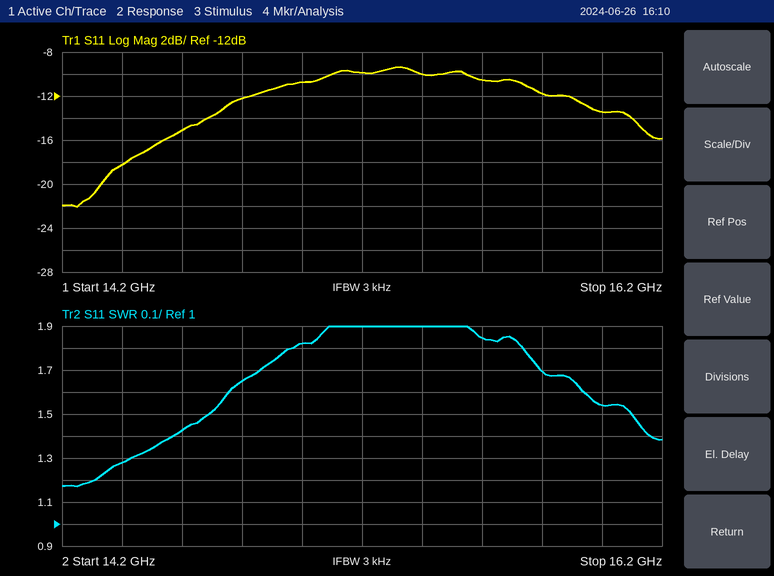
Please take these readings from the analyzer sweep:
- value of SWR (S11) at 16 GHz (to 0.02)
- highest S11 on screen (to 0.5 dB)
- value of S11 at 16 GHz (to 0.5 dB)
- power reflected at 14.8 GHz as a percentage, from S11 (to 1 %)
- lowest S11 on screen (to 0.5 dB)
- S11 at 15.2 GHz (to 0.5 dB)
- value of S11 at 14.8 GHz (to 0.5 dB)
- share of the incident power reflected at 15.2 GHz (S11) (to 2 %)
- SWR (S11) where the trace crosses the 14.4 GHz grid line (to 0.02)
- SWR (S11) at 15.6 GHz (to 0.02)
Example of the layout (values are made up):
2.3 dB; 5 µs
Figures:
1.54; -9.5 dB; -13.5 dB; 6 %; -22.0 dB; -10.0 dB; -12.0 dB; 10 %; 1.28; 1.84
